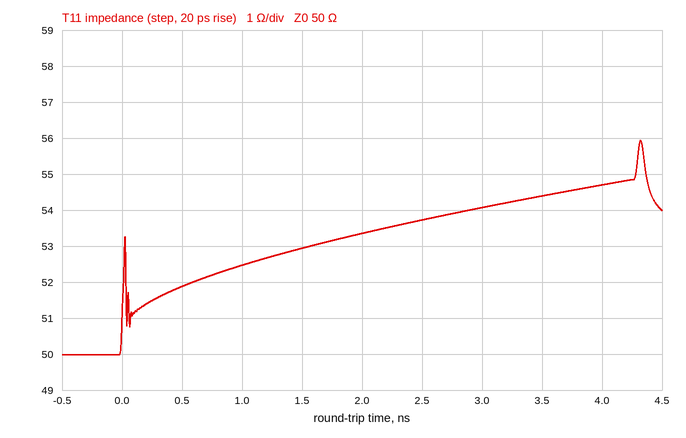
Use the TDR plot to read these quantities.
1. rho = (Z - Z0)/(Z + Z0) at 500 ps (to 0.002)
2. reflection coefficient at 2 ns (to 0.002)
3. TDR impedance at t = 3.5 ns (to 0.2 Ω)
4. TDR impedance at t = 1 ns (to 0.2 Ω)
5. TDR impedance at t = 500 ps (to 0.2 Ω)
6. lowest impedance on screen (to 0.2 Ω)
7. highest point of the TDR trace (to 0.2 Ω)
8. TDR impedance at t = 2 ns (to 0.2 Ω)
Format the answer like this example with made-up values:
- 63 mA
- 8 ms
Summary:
- +0.018
- +0.032
- 54.4 Ω
- 52.4 Ω
- 51.8 Ω
- 50.0 Ω
- 56.0 Ω
- 53.4 Ω
